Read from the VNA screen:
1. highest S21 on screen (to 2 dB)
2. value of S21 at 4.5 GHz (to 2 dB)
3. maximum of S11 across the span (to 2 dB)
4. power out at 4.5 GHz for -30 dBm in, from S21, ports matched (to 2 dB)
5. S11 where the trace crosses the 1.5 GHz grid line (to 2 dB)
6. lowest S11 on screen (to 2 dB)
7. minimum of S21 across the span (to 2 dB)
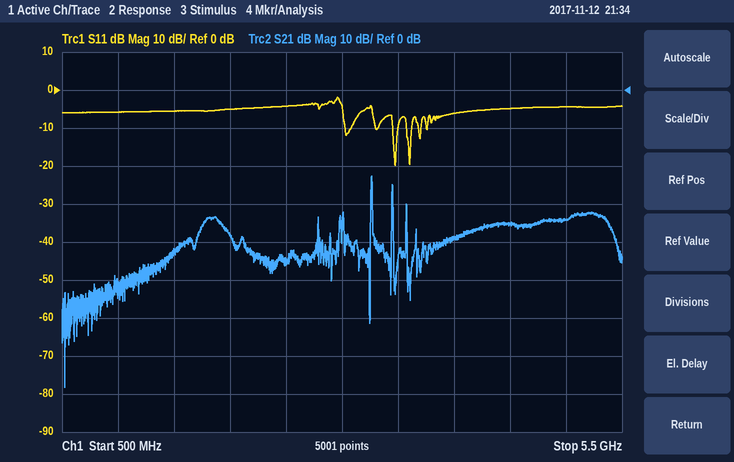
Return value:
-22 dB
-36 dB
-2 dB
-66 dBm
-6 dB
-20 dB
-78 dB
